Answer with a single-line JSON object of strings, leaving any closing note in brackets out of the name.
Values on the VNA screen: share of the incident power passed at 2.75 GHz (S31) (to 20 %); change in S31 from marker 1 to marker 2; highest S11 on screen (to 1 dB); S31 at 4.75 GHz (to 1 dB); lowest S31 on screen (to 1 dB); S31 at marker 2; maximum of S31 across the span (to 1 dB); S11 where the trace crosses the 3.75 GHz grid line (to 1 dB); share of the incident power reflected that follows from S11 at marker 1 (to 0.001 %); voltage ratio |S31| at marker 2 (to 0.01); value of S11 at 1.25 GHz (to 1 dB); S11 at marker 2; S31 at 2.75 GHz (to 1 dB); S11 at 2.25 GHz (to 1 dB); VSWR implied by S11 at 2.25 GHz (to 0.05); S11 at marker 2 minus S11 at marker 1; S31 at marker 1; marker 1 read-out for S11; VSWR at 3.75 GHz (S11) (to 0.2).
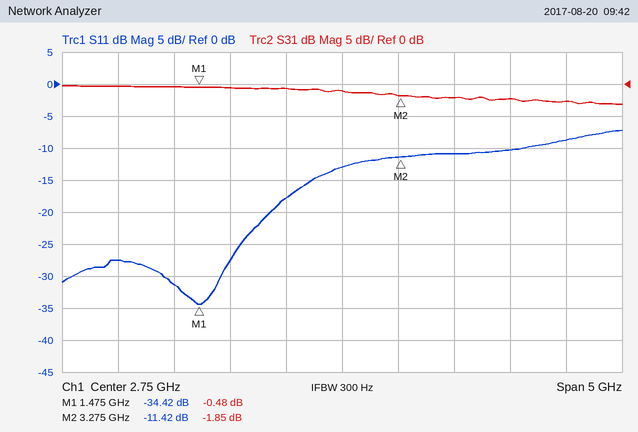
{"share of the incident power passed at 2.75 GHz (S31)": "80 %", "change in S31 from marker 1 to marker 2": "-1.37 dB", "highest S11 on screen": "-7 dB", "S31 at 4.75 GHz": "-3 dB", "lowest S31 on screen": "-3 dB", "S31 at marker 2": "-1.85 dB", "maximum of S31 across the span": "0 dB", "S11 where the trace crosses the 3.75 GHz grid line": "-11 dB", "share of the incident power reflected that follows from S11 at marker 1": "0.036 %", "voltage ratio |S31| at marker 2": "0.81", "value of S11 at 1.25 GHz": "-31 dB", "S11 at marker 2": "-11.42 dB", "S31 at 2.75 GHz": "-1 dB", "S11 at 2.25 GHz": "-18 dB", "VSWR implied by S11 at 2.25 GHz": "1.30", "S11 at marker 2 minus S11 at marker 1": "23.00 dB", "S31 at marker 1": "-0.48 dB", "marker 1 read-out for S11": "-34.42 dB", "VSWR at 3.75 GHz (S11)": "1.8"}
